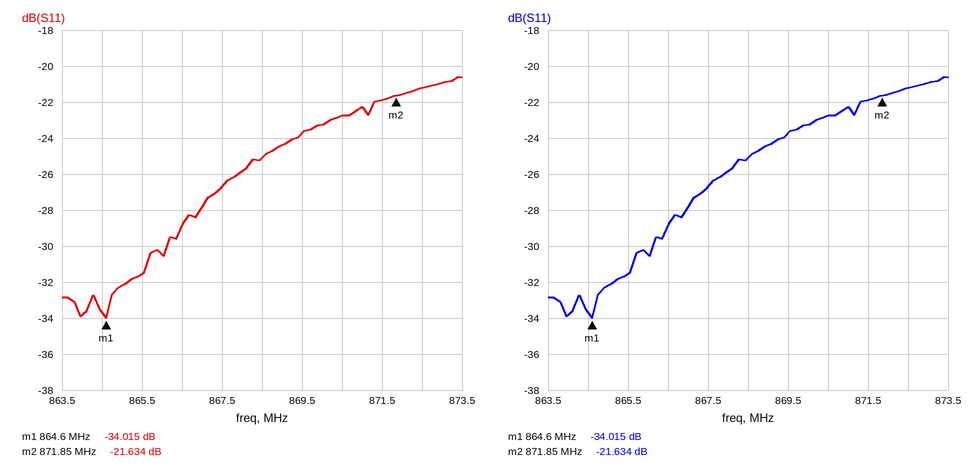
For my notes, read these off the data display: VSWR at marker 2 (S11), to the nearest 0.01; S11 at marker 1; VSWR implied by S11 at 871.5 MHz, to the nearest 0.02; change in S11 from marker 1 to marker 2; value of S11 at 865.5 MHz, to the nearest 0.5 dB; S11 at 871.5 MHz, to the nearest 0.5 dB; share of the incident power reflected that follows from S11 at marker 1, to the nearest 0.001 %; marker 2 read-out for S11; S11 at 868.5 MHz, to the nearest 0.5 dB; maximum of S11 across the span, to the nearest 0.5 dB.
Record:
1.18
-34.015 dB
1.18
12.381 dB
-31.5 dB
-22.0 dB
0.040 %
-21.634 dB
-25.0 dB
-20.5 dB
